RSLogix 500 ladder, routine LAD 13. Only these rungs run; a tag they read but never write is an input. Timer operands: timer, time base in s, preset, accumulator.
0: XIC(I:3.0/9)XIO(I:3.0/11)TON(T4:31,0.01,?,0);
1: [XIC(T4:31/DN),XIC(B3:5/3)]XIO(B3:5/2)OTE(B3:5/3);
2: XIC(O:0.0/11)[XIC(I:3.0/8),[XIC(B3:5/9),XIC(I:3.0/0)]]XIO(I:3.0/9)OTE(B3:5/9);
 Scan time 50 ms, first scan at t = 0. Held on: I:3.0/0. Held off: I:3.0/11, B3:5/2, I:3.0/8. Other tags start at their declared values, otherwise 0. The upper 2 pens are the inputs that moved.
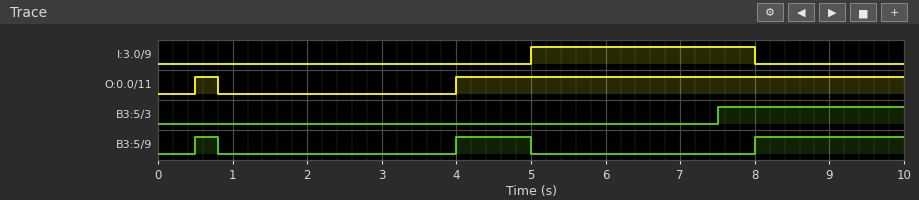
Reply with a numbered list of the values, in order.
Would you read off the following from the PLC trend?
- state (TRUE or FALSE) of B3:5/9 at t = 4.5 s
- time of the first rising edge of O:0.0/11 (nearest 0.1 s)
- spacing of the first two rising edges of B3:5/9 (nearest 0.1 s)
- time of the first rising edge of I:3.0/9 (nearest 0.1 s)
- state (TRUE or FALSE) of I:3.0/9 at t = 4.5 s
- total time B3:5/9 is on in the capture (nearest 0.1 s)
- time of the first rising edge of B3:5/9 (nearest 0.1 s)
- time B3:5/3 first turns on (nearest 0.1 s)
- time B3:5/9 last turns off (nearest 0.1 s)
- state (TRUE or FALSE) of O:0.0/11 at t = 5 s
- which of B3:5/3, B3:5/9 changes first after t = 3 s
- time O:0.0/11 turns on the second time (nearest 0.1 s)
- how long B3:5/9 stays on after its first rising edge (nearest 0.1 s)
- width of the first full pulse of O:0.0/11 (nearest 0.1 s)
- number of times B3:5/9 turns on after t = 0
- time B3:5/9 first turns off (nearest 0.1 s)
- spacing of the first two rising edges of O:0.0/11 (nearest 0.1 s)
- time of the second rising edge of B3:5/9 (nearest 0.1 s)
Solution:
1. TRUE
2. 0.5 s
3. 3.5 s
4. 5.0 s
5. FALSE
6. 3.3 s
7. 0.5 s
8. 7.5 s
9. 5.0 s
10. TRUE
11. B3:5/9
12. 4.0 s
13. 0.3 s
14. 0.3 s
15. 3
16. 0.8 s
17. 3.5 s
18. 4.0 s
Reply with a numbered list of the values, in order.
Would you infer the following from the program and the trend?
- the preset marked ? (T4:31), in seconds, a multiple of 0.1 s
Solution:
1. 2.5 s
